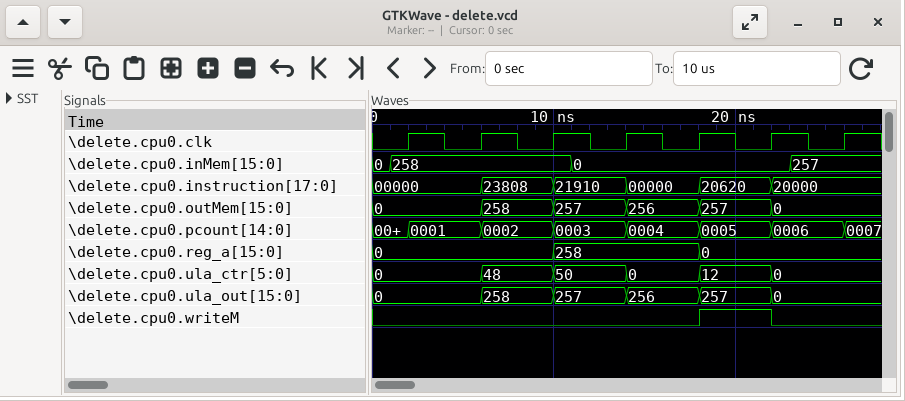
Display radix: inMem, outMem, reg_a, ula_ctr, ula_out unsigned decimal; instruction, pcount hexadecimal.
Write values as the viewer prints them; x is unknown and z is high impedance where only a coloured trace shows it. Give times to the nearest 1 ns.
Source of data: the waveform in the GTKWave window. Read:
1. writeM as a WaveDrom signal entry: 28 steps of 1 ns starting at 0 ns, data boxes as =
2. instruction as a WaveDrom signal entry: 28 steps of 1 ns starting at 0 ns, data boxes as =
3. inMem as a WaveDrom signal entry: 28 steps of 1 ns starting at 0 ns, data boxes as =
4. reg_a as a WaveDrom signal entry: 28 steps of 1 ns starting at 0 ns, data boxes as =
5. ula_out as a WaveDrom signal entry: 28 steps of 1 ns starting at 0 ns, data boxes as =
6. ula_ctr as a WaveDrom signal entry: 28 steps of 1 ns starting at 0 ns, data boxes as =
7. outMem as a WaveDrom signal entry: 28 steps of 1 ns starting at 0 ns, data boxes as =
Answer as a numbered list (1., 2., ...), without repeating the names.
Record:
1. {name: 'writeM', wave: '0.................1...0.....'}
2. {name: 'instruction', wave: '=.....=...=...=...=...=.....', data: '00000 23808 21910 00000 20620 20000'}
3. {name: 'inMem', wave: '==.........=...........=....', data: '0 258 0 257'}
4. {name: 'reg_a', wave: '=.........=.......=.........', data: '0 258 0'}
5. {name: 'ula_out', wave: '=.....=...=...=...=...=.....', data: '0 258 257 256 257 0'}
6. {name: 'ula_ctr', wave: '=.....=...=...=...=...=.....', data: '0 48 50 0 12 0'}
7. {name: 'outMem', wave: '=.....=...=...=...=...=.....', data: '0 258 257 256 257 0'}
